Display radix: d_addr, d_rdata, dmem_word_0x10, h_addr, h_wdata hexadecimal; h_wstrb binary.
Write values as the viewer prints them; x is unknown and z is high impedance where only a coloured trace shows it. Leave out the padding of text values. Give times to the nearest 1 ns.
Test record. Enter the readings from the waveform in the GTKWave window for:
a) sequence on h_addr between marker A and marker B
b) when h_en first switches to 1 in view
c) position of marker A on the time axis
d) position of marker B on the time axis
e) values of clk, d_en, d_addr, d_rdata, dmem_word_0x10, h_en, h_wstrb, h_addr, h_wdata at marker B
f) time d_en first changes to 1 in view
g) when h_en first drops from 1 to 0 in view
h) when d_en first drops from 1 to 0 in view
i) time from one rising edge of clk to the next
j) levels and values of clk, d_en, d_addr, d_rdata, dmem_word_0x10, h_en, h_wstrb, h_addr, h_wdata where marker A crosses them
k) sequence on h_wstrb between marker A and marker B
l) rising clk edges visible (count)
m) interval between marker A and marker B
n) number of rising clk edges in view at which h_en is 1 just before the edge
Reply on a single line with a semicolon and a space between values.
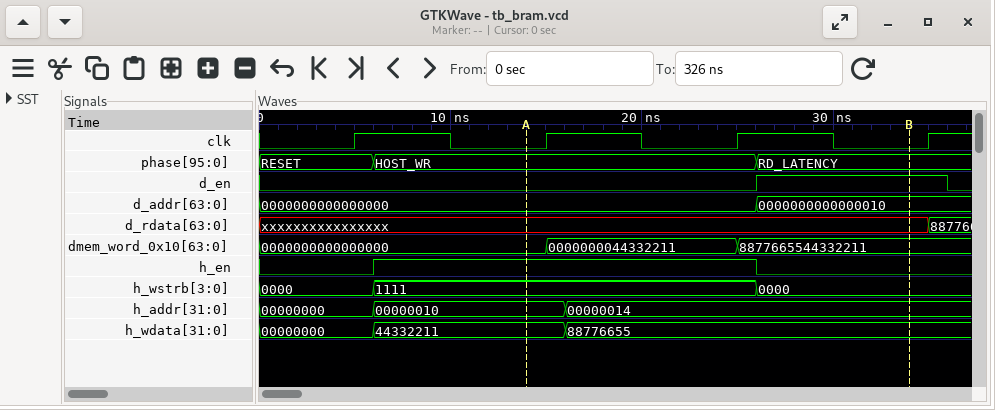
00000010, 00000014; 6 ns; 14 ns; 34 ns; clk=0, d_en=1, d_addr=0000000000000010, d_rdata=xxxxxxxxxxxxxxxx, dmem_word_0x10=8877665544332211, h_en=0, h_wstrb=0000, h_addr=00000014, h_wdata=88776655; 26 ns; 26 ns; 36 ns; 10 ns; clk=0, d_en=0, d_addr=0000000000000000, d_rdata=xxxxxxxxxxxxxxxx, dmem_word_0x10=0000000000000000, h_en=1, h_wstrb=1111, h_addr=00000010, h_wdata=44332211; 1111, 0000; 4; 20 ns; 2
